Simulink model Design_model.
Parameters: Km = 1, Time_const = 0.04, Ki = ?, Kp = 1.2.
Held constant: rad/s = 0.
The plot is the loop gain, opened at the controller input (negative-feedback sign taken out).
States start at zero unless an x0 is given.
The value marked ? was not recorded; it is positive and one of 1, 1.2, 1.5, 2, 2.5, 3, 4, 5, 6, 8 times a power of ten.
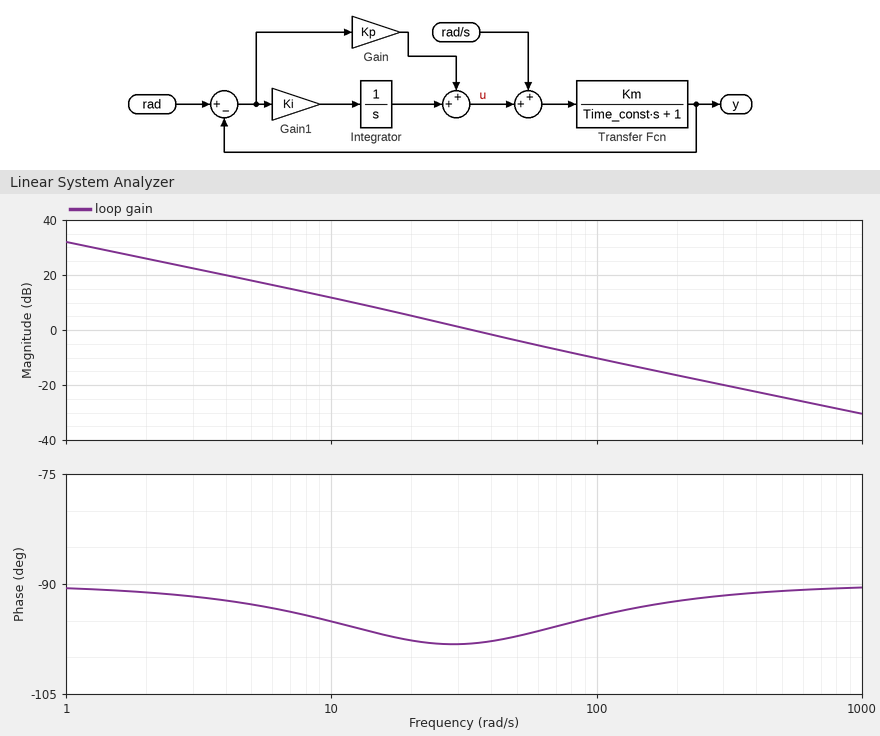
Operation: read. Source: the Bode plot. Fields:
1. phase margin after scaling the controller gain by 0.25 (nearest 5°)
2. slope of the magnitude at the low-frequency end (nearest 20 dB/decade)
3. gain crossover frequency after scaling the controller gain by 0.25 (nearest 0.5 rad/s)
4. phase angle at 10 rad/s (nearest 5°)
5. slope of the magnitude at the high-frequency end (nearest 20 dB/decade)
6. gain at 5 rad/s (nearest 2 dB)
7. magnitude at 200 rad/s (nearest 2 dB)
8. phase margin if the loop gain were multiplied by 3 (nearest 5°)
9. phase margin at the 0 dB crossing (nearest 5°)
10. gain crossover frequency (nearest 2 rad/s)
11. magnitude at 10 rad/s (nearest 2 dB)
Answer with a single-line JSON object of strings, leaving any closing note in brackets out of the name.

{"phase margin after scaling the controller gain by 0.25": "85°", "slope of the magnitude at the low-frequency end": "-20 dB/decade", "gain crossover frequency after scaling the controller gain by 0.25": "9.5 rad/s", "phase angle at 10 rad/s": "-95°", "slope of the magnitude at the high-frequency end": "-20 dB/decade", "gain at 5 rad/s": "18 dB", "magnitude at 200 rad/s": "-16 dB", "phase margin if the loop gain were multiplied by 3": "85°", "phase margin at the 0 dB crossing": "80°", "gain crossover frequency": "34 rad/s", "magnitude at 10 rad/s": "12 dB"}
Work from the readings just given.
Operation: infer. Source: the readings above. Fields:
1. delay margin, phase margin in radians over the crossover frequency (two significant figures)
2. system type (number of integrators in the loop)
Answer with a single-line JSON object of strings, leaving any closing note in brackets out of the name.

{"delay margin, phase margin in radians over the crossover frequency": "0.041 s", "system type": "1"}
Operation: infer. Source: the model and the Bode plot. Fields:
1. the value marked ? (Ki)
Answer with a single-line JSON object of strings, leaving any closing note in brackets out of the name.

{"the value marked ?": "40"}
